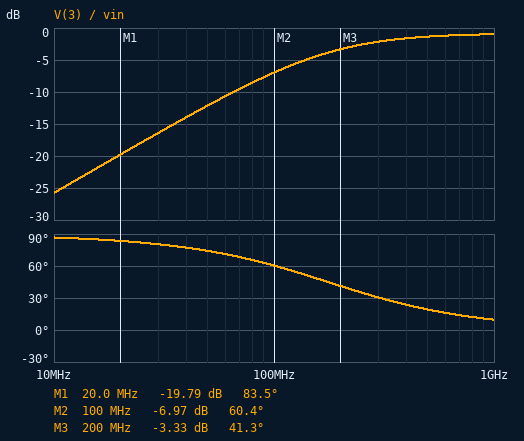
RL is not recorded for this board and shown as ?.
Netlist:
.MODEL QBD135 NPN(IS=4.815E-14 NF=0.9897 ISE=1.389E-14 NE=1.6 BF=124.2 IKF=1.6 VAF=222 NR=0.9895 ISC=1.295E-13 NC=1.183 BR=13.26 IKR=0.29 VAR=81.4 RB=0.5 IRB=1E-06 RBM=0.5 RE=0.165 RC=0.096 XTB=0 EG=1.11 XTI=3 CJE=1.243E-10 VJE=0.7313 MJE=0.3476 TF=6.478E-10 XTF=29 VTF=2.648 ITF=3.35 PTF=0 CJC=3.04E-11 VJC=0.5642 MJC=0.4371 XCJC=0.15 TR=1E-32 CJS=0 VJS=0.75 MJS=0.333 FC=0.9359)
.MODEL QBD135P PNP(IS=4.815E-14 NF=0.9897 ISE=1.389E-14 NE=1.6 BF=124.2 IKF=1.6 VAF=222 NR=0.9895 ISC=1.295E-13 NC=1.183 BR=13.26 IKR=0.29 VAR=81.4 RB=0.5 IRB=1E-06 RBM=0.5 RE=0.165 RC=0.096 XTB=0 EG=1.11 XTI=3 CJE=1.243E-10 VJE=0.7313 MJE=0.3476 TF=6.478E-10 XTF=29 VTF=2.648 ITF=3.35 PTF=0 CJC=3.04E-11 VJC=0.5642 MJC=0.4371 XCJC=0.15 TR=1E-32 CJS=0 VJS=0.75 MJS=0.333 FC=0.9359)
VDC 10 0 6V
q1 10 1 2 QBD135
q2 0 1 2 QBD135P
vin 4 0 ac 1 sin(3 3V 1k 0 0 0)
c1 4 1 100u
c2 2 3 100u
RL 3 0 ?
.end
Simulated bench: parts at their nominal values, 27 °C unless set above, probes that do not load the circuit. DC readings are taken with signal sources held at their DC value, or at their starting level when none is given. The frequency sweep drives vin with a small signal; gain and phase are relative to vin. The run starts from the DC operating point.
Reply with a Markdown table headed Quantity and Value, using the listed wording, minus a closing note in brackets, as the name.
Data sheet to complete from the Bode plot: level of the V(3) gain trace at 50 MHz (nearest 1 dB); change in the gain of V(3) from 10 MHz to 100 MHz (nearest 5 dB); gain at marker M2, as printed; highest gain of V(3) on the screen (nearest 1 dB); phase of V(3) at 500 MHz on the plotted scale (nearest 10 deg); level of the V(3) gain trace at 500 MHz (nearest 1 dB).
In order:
| Quantity | Value |
|---|---|
| level of the V(3) gain trace at 50 MHz | -12 dB |
| change in the gain of V(3) from 10 MHz to 100 MHz | 20 dB |
| gain at marker M2, as printed | -6.97 dB |
| highest gain of V(3) on the screen | -1 dB |
| phase of V(3) at 500 MHz on the plotted scale | 20 deg |
| level of the V(3) gain trace at 500 MHz | -1 dB |
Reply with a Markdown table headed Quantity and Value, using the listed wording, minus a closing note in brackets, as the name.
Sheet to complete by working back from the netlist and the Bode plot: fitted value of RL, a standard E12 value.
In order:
| Quantity | Value |
|---|---|
| fitted value of RL, a standard E12 value | 3.3 Ω |
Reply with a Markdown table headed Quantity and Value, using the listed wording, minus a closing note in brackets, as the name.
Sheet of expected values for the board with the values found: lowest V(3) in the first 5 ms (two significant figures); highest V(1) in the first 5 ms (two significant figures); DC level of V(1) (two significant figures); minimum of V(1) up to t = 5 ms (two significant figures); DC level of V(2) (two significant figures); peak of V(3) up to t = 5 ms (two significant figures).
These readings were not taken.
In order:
| Quantity | Value |
|---|---|
| lowest V(3) in the first 5 ms | -2.1 V |
| highest V(1) in the first 5 ms | 5.3 V |
| DC level of V(1) | 2.0 V |
| minimum of V(1) up to t = 5 ms | -890 mV |
| DC level of V(2) | 2.0 V |
| peak of V(3) up to t = 5 ms | 2.0 V |
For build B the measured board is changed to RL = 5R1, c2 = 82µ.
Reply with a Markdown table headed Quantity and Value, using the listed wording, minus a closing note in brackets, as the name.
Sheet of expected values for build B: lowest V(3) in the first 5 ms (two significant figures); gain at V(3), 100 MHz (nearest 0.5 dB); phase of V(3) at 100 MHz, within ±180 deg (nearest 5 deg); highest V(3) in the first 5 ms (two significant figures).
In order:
| Quantity | Value |
|---|---|
| lowest V(3) in the first 5 ms | -2.2 V |
| gain at V(3), 100 MHz | -4.5 dB |
| phase of V(3) at 100 MHz, within ±180 deg | 50 deg |
| highest V(3) in the first 5 ms | 2.1 V |
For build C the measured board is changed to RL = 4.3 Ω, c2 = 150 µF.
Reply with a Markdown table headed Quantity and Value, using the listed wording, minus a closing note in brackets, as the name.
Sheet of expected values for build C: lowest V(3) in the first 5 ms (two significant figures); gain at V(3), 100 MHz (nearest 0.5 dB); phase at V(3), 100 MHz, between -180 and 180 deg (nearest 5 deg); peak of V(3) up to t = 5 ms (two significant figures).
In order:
| Quantity | Value |
|---|---|
| lowest V(3) in the first 5 ms | -2.2 V |
| gain at V(3), 100 MHz | -5.5 dB |
| phase at V(3), 100 MHz, between -180 and 180 deg | 55 deg |
| peak of V(3) up to t = 5 ms | 2.1 V |
